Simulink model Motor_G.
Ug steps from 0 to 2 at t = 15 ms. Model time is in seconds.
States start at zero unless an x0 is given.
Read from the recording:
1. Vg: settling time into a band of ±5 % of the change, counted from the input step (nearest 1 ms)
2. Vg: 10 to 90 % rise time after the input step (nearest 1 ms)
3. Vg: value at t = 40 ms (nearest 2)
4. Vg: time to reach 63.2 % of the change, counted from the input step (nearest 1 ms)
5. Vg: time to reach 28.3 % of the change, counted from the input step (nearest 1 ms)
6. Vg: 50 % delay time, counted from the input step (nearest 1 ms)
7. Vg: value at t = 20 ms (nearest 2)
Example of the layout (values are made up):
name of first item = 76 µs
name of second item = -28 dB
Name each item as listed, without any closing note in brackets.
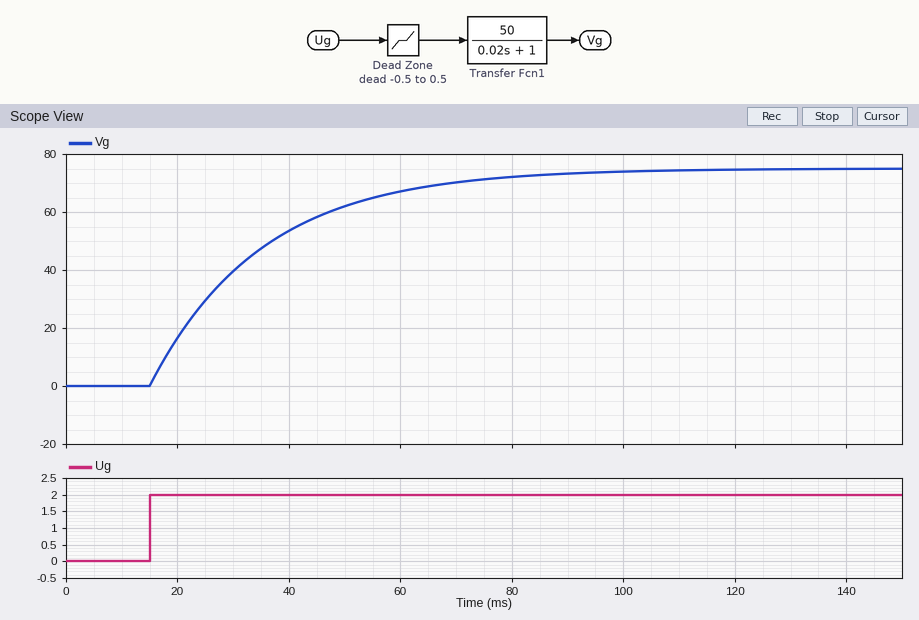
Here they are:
Vg: settling time into a band of ±5 % of the change, counted from the input step = 60 ms
Vg: 10 to 90 % rise time after the input step = 44 ms
Vg: value at t = 40 ms = 54
Vg: time to reach 63.2 % of the change, counted from the input step = 20 ms
Vg: time to reach 28.3 % of the change, counted from the input step = 7 ms
Vg: 50 % delay time, counted from the input step = 14 ms
Vg: value at t = 20 ms = 16
